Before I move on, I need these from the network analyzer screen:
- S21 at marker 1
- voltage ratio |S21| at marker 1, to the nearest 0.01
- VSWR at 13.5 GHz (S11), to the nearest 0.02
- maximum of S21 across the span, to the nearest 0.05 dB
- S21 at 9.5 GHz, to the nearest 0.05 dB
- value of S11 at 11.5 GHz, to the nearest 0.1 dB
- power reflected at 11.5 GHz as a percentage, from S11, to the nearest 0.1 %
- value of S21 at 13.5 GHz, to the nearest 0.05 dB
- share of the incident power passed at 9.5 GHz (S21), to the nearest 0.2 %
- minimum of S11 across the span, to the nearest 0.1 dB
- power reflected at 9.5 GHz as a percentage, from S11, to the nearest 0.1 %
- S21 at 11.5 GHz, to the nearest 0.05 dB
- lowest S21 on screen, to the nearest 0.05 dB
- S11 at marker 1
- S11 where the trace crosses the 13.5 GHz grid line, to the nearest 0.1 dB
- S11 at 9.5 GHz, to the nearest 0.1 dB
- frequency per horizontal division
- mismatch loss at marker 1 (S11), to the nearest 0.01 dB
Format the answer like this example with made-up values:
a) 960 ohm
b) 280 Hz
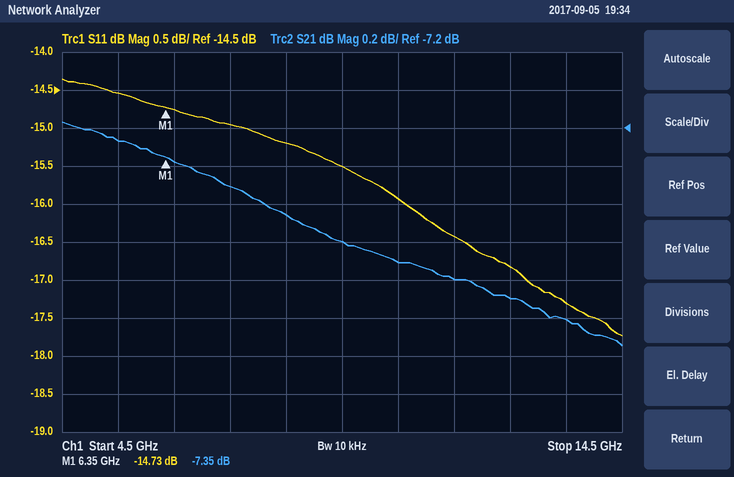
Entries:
a) -7.35 dB
b) 0.43
c) 1.32
d) -7.15 dB
e) -7.80 dB
f) -16.4 dB
g) 2.3 %
h) -8.20 dB
i) 16.6 %
j) -17.7 dB
k) 2.8 %
l) -8.00 dB
m) -8.35 dB
n) -14.73 dB
o) -17.3 dB
p) -15.5 dB
q) 1 GHz
r) 0.15 dB
